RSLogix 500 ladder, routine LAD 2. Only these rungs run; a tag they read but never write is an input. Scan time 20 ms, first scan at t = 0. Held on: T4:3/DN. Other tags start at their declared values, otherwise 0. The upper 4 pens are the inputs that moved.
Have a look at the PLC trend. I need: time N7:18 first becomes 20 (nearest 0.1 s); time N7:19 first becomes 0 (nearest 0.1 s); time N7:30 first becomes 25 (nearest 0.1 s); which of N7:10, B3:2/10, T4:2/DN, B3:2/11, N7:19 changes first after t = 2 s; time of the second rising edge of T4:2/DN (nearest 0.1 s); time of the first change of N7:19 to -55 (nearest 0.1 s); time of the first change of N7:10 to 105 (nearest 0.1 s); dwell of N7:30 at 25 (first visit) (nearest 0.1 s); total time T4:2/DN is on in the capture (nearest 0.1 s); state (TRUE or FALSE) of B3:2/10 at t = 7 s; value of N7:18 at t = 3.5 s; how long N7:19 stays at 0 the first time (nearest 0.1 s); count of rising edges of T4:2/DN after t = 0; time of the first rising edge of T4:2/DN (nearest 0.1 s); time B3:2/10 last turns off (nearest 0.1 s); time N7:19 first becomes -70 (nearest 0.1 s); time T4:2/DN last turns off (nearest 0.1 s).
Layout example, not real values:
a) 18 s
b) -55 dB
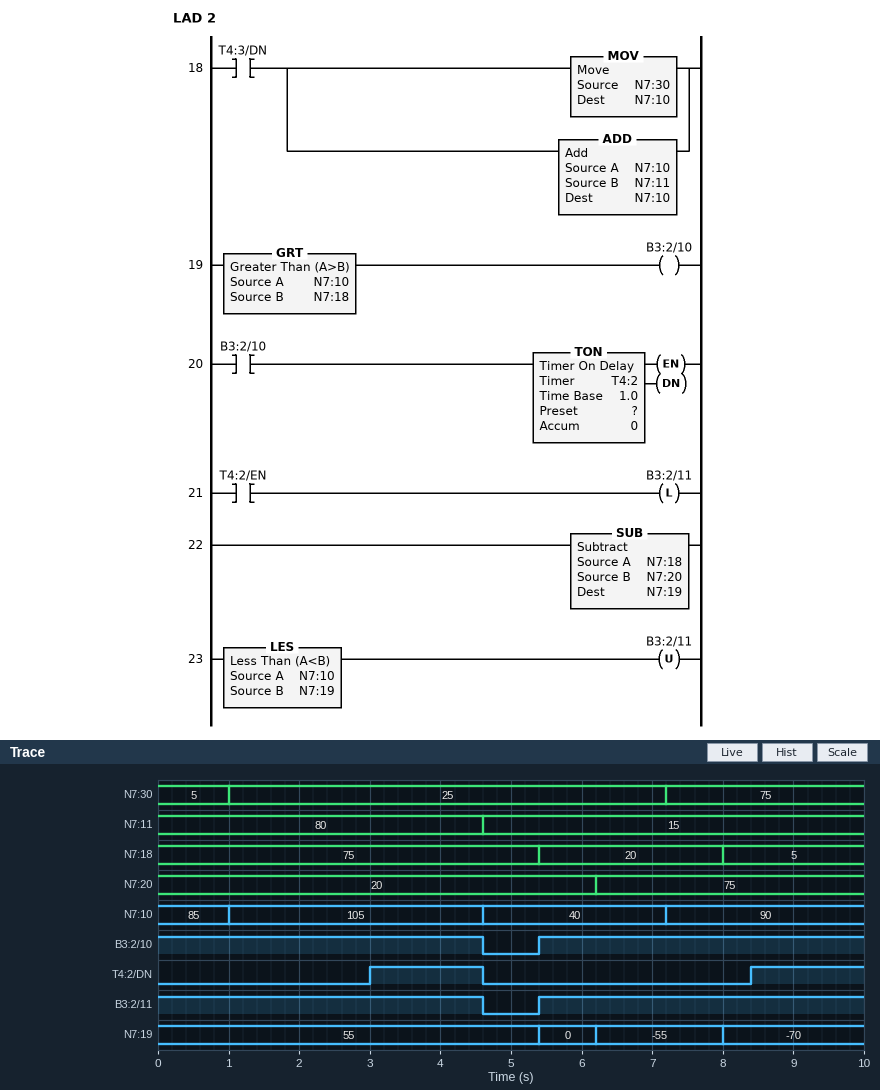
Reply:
a) 5.4 s
b) 5.4 s
c) 1.0 s
d) T4:2/DN
e) 8.4 s
f) 6.2 s
g) 1.0 s
h) 6.2 s
i) 3.2 s
j) TRUE
k) 75
l) 0.8 s
m) 2
n) 3.0 s
o) 4.6 s
p) 8.0 s
q) 4.6 s
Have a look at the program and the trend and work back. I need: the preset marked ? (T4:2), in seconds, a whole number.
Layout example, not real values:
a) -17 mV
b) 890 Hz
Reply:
a) 3 s
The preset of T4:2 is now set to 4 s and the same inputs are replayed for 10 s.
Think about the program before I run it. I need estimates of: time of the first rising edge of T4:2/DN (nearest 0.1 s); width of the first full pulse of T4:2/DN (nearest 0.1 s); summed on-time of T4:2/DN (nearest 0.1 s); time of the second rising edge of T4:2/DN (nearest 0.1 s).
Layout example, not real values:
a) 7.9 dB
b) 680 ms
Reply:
a) 4.0 s
b) 0.6 s
c) 1.2 s
d) 9.4 s
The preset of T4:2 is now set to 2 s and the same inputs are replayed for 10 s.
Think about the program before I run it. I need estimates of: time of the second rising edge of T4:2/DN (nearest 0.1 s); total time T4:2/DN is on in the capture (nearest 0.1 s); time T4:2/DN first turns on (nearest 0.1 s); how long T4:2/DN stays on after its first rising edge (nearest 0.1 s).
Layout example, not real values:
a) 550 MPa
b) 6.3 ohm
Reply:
a) 7.4 s
b) 5.2 s
c) 2.0 s
d) 2.6 s
